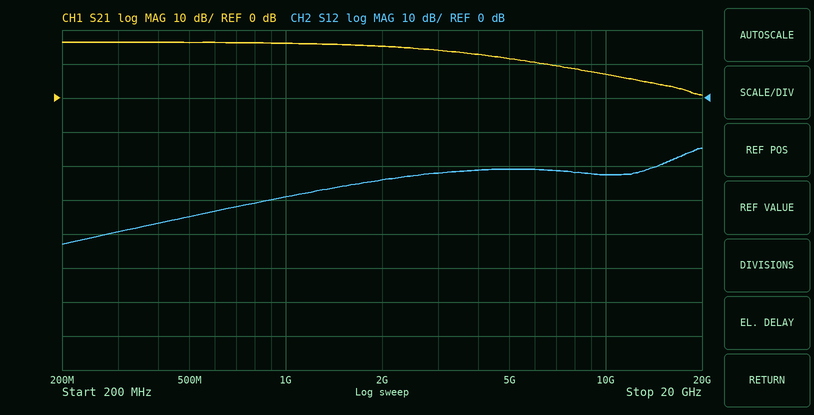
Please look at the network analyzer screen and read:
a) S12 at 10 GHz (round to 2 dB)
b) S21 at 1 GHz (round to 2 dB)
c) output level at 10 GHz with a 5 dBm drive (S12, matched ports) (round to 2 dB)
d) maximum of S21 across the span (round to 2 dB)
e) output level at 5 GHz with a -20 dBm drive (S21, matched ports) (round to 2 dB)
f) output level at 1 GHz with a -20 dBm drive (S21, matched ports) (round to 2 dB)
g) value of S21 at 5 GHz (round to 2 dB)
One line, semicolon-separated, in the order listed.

-22 dB; 16 dB; -18 dBm; 16 dB; -8 dBm; -4 dBm; 12 dB
